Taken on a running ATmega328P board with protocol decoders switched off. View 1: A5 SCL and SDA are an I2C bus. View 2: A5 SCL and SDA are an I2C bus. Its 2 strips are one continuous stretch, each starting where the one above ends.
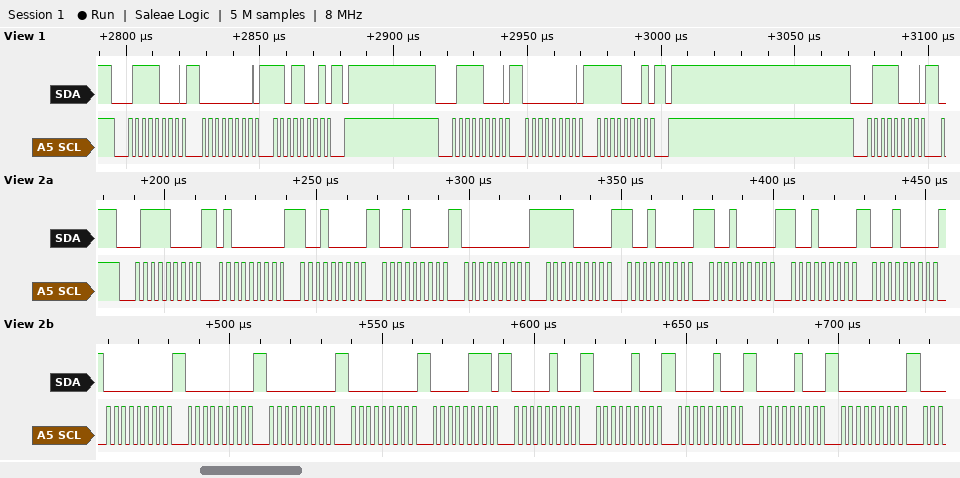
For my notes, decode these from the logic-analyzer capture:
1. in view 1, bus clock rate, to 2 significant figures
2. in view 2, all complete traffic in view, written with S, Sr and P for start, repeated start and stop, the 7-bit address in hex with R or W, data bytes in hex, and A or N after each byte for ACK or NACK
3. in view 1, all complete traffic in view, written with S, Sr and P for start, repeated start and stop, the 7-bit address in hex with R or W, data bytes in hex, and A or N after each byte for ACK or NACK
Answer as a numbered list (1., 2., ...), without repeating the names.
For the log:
1. 400 kHz
2. S 3CW A 40 A 90 A 10 A 00 A F0 A 90 A 90 A 90 A 10 A 00 A 00 A 00 A 00 A 07 A 04 A 04 A 04 A 04 A 00 A
3. S 3CW A 00 A D9 A P S 3CW A 00 A F1 A P S 3CW A
